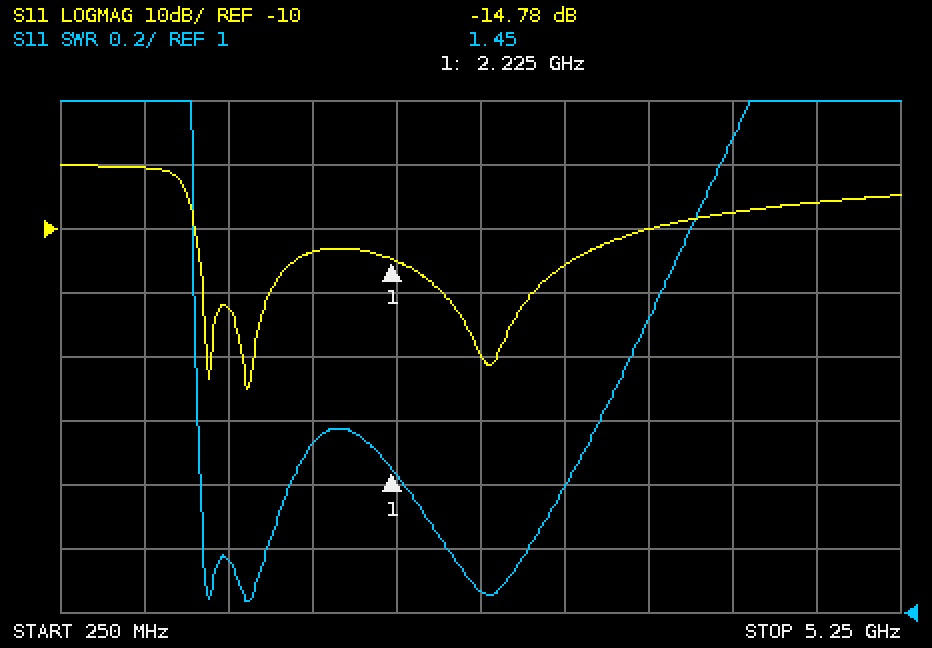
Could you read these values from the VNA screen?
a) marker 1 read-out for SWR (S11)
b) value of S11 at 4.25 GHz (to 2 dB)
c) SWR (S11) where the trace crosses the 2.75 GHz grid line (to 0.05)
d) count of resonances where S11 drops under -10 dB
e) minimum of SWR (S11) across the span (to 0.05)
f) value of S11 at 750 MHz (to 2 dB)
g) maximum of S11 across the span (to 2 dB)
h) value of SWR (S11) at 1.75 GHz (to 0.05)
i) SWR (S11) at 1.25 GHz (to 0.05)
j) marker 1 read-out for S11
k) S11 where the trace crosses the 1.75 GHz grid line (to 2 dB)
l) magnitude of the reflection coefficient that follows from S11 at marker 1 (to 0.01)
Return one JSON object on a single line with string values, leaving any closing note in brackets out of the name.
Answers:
{"marker 1 read-out for SWR": "1.45", "value of S11 at 4.25 GHz": "-8 dB", "SWR (S11) where the trace crosses the 2.75 GHz grid line": "1.05", "count of resonances where S11 drops under -10 dB": "3", "minimum of SWR (S11) across the span": "1.05", "value of S11 at 750 MHz": "0 dB", "maximum of S11 across the span": "0 dB", "value of SWR (S11) at 1.75 GHz": "1.55", "SWR (S11) at 1.25 GHz": "1.15", "marker 1 read-out for S11": "-14.78 dB", "S11 where the trace crosses the 1.75 GHz grid line": "-14 dB", "magnitude of the reflection coefficient that follows from S11 at marker 1": "0.18"}
